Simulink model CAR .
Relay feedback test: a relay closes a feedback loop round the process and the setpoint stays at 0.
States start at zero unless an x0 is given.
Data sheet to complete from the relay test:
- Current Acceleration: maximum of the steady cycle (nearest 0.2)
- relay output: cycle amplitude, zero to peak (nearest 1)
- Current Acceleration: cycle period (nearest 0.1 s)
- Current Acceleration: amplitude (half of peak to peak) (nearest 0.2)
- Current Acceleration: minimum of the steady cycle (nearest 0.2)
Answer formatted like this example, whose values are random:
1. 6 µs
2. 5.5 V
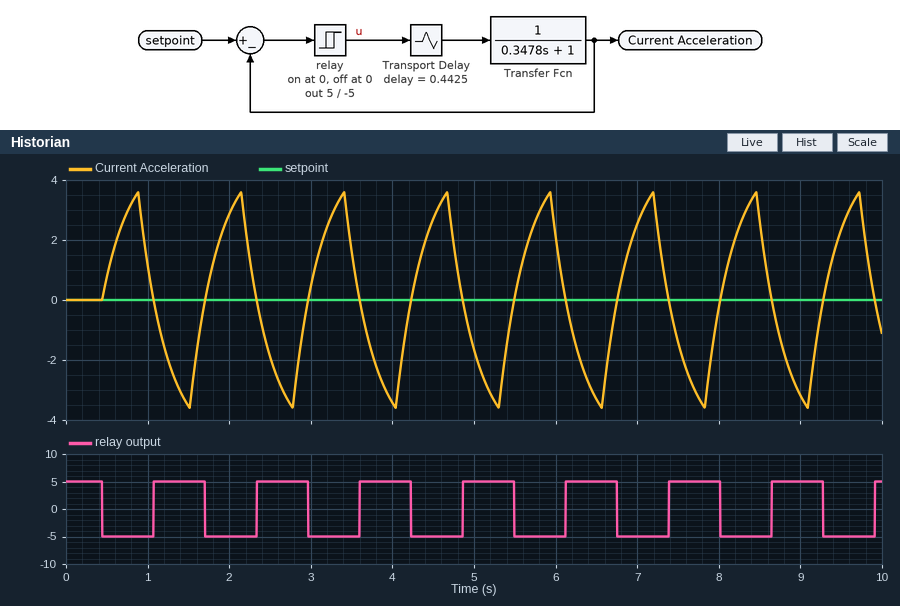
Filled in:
1. 3.6
2. 5
3. 1.3 s
4. 3.6
5. -3.6
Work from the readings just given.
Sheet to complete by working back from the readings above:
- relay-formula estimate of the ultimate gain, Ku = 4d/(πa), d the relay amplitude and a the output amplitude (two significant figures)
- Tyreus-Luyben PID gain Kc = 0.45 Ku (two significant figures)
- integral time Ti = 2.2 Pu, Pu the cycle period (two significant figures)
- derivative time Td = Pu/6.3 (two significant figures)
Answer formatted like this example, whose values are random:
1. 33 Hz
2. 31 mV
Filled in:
1. 1.8
2. 0.81
3. 2.9 s
4. 0.21 s
